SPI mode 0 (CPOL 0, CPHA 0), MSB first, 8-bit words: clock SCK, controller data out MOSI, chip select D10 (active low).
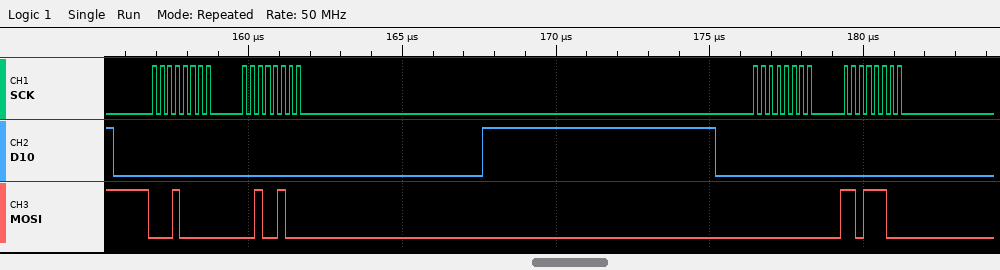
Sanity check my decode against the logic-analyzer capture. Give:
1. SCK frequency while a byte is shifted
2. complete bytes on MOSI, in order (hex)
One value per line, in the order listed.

4 MHz
0x10 0x24 0x00 0xDC
